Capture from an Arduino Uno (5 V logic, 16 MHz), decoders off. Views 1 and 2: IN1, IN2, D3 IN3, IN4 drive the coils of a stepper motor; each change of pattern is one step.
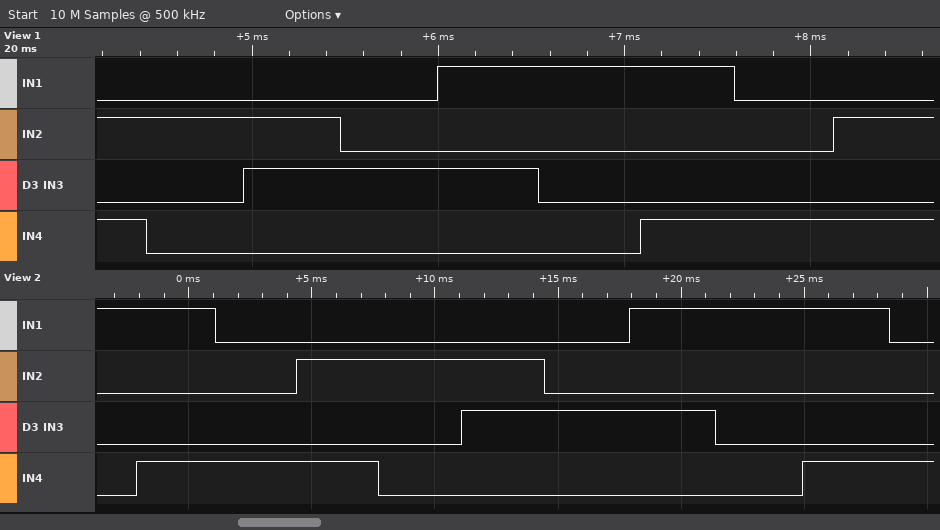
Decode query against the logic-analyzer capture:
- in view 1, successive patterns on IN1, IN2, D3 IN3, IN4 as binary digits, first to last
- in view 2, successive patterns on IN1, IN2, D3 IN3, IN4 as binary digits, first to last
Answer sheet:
0101 0100 0110 0010 1010 1000 1001 0001 0101
1000 1001 0001 0101 0100 0110 0010 1010 1000 1001 0001
